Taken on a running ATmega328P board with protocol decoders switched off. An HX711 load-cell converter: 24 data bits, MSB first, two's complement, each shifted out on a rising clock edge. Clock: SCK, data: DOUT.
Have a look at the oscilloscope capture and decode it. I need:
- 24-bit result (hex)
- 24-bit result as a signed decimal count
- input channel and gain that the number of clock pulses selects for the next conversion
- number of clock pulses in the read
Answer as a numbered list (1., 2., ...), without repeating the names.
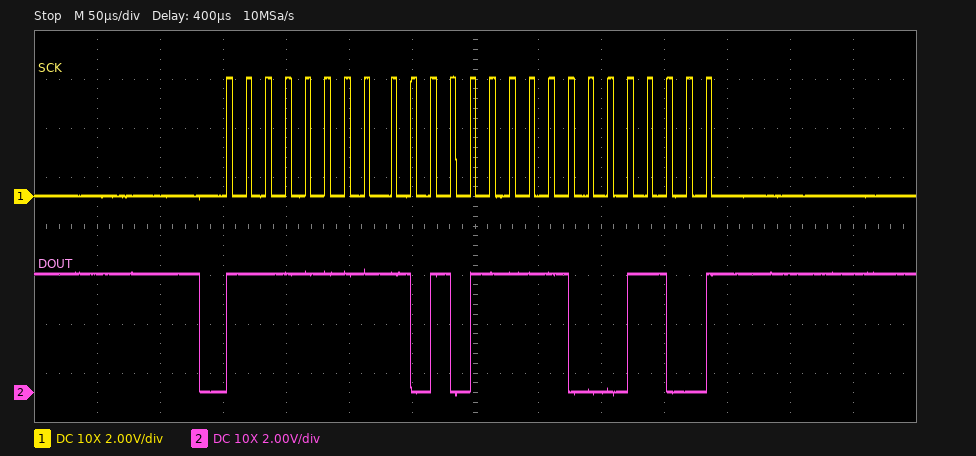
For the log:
1. 0xFFAF8C
2. -20596
3. channel A, gain 128
4. 25
